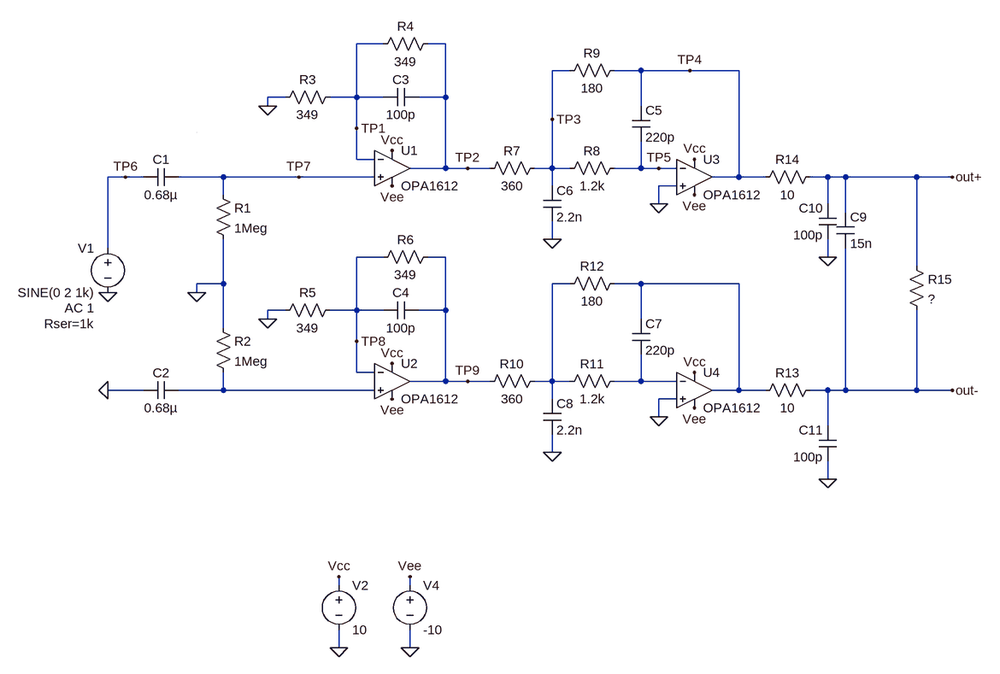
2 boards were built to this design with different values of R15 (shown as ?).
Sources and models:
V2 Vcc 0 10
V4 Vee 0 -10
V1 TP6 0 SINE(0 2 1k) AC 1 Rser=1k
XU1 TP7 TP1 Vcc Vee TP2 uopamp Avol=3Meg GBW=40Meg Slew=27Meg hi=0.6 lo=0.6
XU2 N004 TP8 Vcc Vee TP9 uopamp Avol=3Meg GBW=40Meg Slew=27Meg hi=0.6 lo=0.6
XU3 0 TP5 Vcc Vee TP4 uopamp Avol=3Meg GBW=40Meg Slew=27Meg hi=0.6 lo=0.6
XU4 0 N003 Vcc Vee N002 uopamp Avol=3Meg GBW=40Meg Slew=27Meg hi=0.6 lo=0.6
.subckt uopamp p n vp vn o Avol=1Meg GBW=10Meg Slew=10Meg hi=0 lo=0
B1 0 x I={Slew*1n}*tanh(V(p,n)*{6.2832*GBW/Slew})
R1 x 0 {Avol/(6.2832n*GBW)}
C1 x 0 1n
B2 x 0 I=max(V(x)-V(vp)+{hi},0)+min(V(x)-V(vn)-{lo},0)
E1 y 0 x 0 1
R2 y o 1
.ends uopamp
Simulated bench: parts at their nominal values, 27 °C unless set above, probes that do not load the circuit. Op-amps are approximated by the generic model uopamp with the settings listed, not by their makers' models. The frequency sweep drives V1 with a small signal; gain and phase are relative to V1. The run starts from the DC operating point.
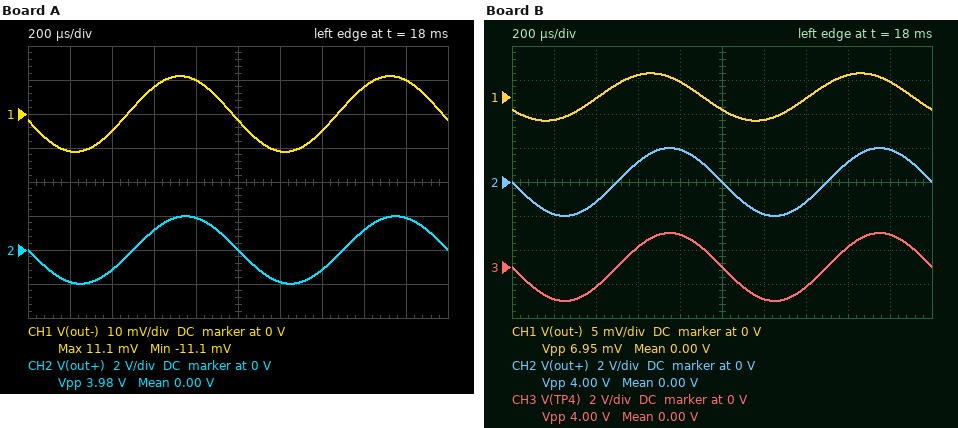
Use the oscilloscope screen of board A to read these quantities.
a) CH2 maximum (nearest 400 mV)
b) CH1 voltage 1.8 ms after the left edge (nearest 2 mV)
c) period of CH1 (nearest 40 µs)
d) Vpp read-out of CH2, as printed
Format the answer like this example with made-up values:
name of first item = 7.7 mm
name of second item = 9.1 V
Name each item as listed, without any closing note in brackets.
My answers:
CH2 maximum = 2.0 V
CH1 voltage 1.8 ms after the left edge = 10 mV
period of CH1 = 1.00 ms
Vpp read-out of CH2, as printed = 3.98 V
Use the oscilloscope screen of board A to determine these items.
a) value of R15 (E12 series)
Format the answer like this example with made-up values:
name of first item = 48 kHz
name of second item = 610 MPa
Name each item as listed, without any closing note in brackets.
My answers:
value of R15 = 1.8 kΩ
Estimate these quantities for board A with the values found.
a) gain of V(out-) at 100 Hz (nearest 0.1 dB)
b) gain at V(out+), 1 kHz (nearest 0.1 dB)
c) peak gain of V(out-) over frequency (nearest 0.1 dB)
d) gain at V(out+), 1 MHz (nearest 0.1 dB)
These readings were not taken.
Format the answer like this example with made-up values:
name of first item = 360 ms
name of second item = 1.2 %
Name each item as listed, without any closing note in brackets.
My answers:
gain of V(out-) at 100 Hz = -45.2 dB
gain at V(out+), 1 kHz = -0.1 dB
peak gain of V(out-) over frequency = -11.7 dB
gain at V(out+), 1 MHz = -16.5 dB
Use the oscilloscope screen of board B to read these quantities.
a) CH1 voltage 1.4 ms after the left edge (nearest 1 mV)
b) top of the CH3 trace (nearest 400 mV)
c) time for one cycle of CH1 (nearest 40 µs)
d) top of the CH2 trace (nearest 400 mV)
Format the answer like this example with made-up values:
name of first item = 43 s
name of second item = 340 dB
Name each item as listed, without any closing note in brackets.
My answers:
CH1 voltage 1.4 ms after the left edge = 0 V
top of the CH3 trace = 2.0 V
time for one cycle of CH1 = 1.00 ms
top of the CH2 trace = 2.0 V
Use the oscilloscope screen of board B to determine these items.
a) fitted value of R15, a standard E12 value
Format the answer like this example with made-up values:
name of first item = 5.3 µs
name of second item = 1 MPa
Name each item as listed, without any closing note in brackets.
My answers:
fitted value of R15, a standard E12 value = 6.8 kΩ
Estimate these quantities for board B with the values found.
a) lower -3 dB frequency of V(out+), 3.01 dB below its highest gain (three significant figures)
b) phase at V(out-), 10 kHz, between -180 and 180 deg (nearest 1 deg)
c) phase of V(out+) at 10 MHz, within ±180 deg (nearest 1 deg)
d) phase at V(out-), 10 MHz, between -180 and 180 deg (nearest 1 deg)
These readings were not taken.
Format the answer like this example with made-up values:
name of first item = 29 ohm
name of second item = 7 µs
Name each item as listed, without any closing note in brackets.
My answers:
lower -3 dB frequency of V(out+), 3.01 dB below its highest gain = 234 mHz
phase at V(out-), 10 kHz, between -180 and 180 deg = -102 deg
phase of V(out+) at 10 MHz, within ±180 deg = -50 deg
phase at V(out-), 10 MHz, between -180 and 180 deg = -44 deg
